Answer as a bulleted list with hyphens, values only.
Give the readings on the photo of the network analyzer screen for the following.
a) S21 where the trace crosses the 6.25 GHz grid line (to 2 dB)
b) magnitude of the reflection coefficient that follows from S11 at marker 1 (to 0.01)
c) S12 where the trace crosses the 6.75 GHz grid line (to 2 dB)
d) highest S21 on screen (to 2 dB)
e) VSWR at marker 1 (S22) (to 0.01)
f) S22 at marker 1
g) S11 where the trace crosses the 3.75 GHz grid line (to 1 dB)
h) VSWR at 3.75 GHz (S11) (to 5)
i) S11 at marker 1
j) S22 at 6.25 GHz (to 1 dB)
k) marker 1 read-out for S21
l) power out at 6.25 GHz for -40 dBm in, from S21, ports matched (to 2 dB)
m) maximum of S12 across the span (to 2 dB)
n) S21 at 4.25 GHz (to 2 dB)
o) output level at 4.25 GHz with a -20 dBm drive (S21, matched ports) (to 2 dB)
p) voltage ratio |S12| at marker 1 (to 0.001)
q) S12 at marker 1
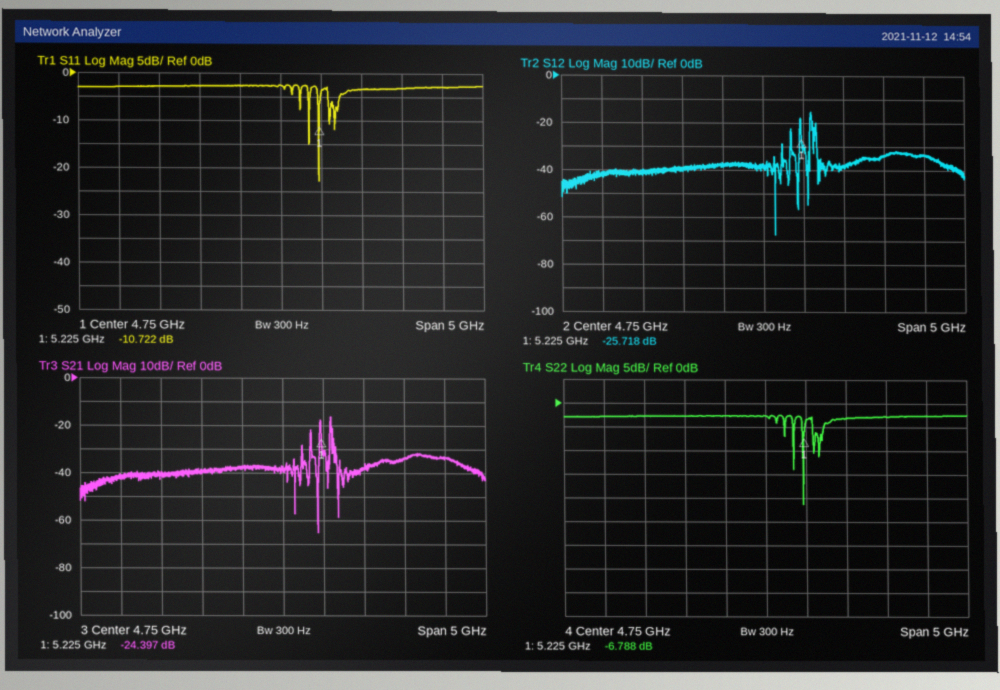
- -34 dB
- 0.29
- -34 dB
- -16 dB
- 2.69
- -6.788 dB
- -3 dB
- 5
- -10.722 dB
- -3 dB
- -24.397 dB
- -74 dBm
- -16 dB
- -38 dB
- -58 dBm
- 0.052
- -25.718 dB
